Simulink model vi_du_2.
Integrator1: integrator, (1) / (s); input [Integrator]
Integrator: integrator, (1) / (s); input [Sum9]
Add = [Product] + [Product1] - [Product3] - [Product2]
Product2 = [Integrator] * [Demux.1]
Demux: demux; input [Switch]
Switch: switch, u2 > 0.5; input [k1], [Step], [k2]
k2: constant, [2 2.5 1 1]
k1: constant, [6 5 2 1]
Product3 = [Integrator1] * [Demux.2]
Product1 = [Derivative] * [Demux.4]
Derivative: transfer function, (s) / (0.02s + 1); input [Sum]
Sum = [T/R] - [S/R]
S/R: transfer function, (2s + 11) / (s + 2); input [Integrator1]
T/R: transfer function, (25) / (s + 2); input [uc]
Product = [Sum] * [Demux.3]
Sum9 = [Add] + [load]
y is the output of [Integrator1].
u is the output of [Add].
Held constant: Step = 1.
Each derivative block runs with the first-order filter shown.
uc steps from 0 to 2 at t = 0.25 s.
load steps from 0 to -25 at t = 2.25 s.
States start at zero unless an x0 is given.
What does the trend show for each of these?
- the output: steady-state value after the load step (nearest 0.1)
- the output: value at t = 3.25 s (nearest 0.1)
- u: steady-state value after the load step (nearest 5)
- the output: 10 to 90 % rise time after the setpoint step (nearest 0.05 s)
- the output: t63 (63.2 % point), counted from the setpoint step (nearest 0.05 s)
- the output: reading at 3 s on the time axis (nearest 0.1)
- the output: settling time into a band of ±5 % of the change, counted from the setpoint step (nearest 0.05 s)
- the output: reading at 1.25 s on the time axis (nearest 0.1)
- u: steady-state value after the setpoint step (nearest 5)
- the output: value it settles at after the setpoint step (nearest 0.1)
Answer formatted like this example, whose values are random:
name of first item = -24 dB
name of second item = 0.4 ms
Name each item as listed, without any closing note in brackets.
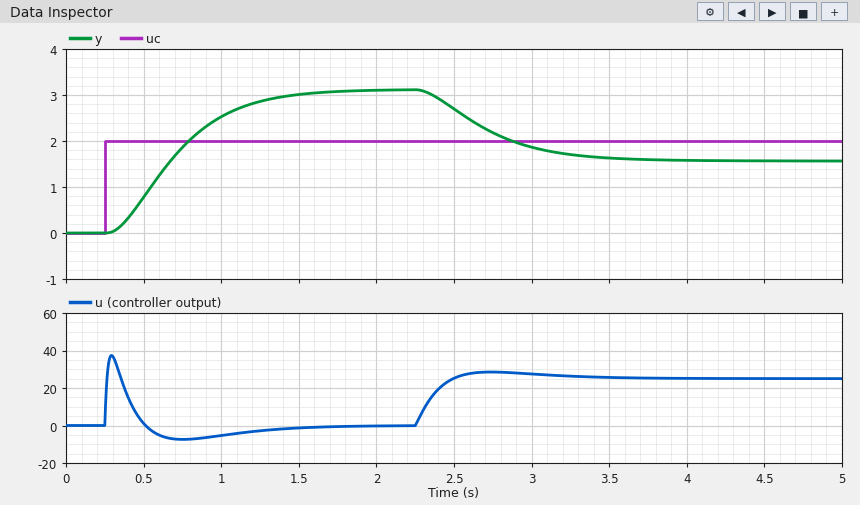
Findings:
the output: steady-state value after the load step = 1.6
the output: value at t = 3.25 s = 1.7
u: steady-state value after the load step = 25
the output: 10 to 90 % rise time after the setpoint step = 0.80 s
the output: t63 (63.2 % point), counted from the setpoint step = 0.55 s
the output: reading at 3 s on the time axis = 1.9
the output: settling time into a band of ±5 % of the change, counted from the setpoint step = 1.15 s
the output: reading at 1.25 s on the time axis = 2.9
u: steady-state value after the setpoint step = 0
the output: value it settles at after the setpoint step = 3.1
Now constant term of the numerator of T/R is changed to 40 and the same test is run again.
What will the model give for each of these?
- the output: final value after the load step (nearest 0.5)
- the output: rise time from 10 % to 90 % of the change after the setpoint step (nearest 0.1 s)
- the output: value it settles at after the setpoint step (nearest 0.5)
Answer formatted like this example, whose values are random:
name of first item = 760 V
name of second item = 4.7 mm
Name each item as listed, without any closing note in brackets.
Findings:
the output: final value after the load step = 3.5
the output: rise time from 10 % to 90 % of the change after the setpoint step = 0.8 s
the output: value it settles at after the setpoint step = 5.0
